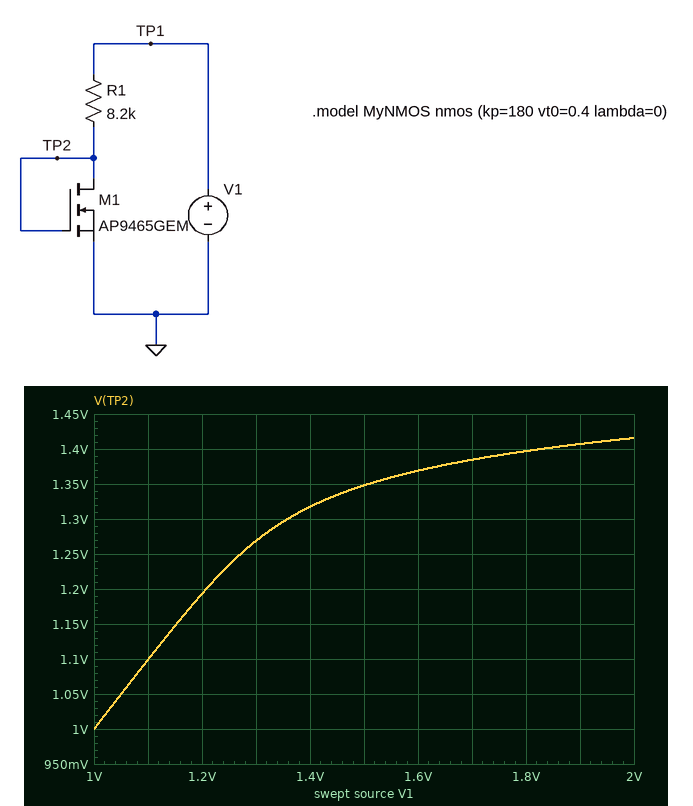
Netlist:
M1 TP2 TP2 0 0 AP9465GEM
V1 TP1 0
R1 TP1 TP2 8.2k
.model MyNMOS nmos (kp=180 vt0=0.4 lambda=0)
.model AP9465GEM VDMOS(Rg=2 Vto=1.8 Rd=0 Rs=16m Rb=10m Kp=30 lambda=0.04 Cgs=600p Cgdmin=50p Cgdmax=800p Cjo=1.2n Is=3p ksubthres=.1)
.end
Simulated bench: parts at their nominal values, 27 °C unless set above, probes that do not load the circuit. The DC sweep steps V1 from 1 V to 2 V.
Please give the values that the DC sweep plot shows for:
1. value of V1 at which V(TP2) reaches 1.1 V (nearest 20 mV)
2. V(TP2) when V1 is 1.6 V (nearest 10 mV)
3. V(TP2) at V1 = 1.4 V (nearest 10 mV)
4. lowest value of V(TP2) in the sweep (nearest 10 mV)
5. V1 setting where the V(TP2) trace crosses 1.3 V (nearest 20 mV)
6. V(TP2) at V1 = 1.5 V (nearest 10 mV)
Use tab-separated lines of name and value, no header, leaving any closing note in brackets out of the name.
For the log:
value of V1 at which V(TP2) reaches 1.1 V	1.10 V
V(TP2) when V1 is 1.6 V	1.37 V
V(TP2) at V1 = 1.4 V	1.32 V
lowest value of V(TP2) in the sweep	1.00 V
V1 setting where the V(TP2) trace crosses 1.3 V	1.36 V
V(TP2) at V1 = 1.5 V	1.35 V
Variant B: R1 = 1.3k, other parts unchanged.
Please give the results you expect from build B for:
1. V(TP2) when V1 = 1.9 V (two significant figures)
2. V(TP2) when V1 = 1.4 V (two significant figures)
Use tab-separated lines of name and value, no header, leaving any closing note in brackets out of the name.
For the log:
V(TP2) when V1 = 1.9 V	1.5 V
V(TP2) when V1 = 1.4 V	1.4 V
